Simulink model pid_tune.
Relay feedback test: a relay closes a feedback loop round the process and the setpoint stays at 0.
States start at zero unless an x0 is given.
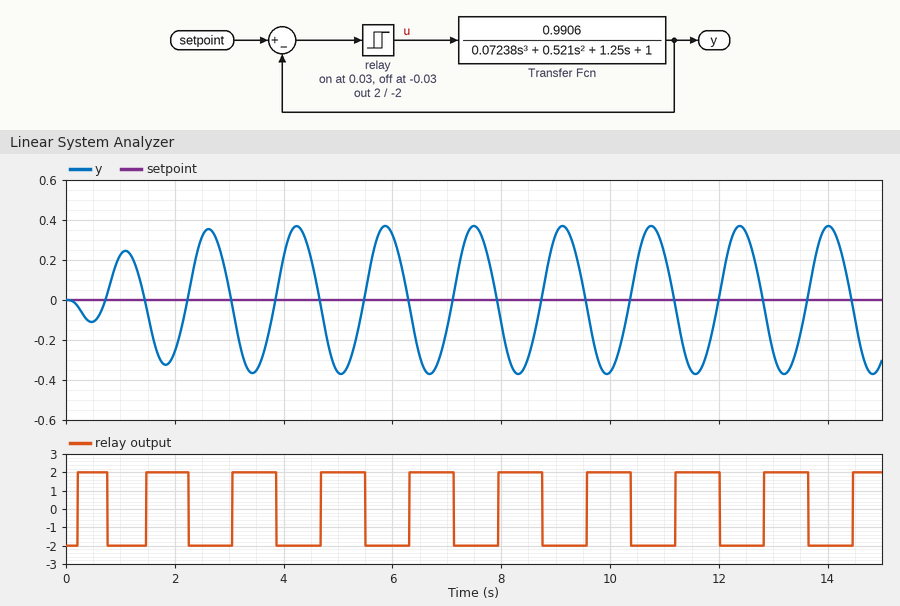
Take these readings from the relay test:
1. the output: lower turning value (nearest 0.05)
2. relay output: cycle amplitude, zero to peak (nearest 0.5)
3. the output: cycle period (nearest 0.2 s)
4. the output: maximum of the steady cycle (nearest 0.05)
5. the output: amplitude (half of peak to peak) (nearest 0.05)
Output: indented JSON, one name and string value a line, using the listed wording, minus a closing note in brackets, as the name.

{
  "the output: lower turning value": "-0.35",
  "relay output: cycle amplitude, zero to peak": "2.0",
  "the output: cycle period": "1.6 s",
  "the output: maximum of the steady cycle": "0.35",
  "the output: amplitude (half of peak to peak)": "0.35"
}
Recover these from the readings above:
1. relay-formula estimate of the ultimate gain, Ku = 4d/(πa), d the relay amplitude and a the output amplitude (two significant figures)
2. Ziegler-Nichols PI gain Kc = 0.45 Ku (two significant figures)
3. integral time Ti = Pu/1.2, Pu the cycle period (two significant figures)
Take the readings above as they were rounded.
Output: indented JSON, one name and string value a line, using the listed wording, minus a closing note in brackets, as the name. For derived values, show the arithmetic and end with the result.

{
  "relay-formula estimate of the ultimate gain, Ku = 4d/(πa), d the relay amplitude and a the output amplitude": "4 × 2 / (π × 0.35) = 7.3",
  "Ziegler-Nichols PI gain Kc = 0.45 Ku": "0.45 × 7.3 = 3.3",
  "integral time Ti = Pu/1.2, Pu the cycle period": "1.6 / 1.2 = 1.3 s"
}
